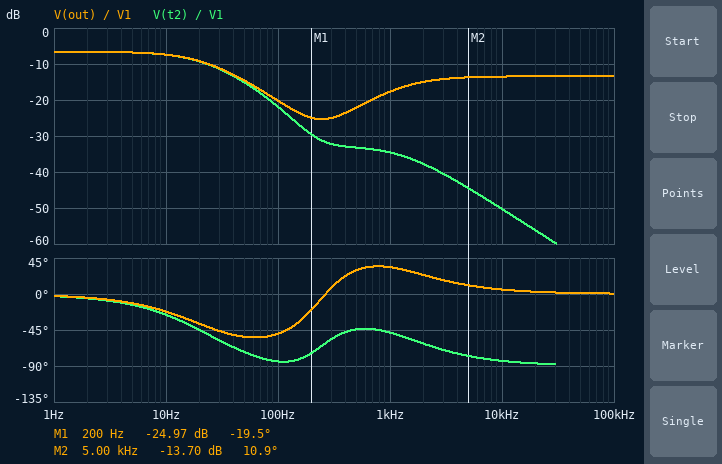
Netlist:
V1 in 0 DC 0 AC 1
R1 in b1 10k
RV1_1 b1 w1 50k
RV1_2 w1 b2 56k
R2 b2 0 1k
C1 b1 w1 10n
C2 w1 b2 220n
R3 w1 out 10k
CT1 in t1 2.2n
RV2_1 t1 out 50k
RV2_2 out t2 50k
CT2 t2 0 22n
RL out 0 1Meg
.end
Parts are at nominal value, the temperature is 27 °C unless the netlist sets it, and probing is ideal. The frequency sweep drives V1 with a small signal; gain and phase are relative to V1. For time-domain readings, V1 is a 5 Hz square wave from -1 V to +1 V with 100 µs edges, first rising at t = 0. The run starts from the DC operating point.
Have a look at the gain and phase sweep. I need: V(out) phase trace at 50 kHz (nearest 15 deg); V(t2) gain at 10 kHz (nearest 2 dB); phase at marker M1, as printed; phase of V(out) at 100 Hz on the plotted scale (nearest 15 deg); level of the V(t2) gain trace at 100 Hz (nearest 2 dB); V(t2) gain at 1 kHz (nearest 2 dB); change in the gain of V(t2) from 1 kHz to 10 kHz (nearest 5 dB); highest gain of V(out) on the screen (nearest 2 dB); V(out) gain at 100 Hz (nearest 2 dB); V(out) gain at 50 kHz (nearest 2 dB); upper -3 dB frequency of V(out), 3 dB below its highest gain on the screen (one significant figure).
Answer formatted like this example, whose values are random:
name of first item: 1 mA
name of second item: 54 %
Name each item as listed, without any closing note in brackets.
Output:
V(out) phase trace at 50 kHz: 0 deg
V(t2) gain at 10 kHz: -50 dB
phase at marker M1, as printed: -19.5 deg
phase of V(out) at 100 Hz on the plotted scale: -45 deg
level of the V(t2) gain trace at 100 Hz: -22 dB
V(t2) gain at 1 kHz: -34 dB
change in the gain of V(t2) from 1 kHz to 10 kHz: -15 dB
highest gain of V(out) on the screen: -6 dB
V(out) gain at 100 Hz: -20 dB
V(out) gain at 50 kHz: -14 dB
upper -3 dB frequency of V(out), 3 dB below its highest gain on the screen: 20 Hz
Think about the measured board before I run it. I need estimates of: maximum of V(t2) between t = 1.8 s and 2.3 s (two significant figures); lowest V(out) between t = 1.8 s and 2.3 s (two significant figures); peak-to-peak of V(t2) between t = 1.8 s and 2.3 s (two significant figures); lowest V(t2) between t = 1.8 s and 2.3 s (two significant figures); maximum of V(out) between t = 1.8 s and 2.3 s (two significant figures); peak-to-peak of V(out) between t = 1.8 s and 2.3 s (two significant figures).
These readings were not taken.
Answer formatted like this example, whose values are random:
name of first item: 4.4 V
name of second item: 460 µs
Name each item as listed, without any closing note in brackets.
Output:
maximum of V(t2) between t = 1.8 s and 2.3 s: 470 mV
lowest V(out) between t = 1.8 s and 2.3 s: -470 mV
peak-to-peak of V(t2) between t = 1.8 s and 2.3 s: 940 mV
lowest V(t2) between t = 1.8 s and 2.3 s: -470 mV
maximum of V(out) between t = 1.8 s and 2.3 s: 470 mV
peak-to-peak of V(out) between t = 1.8 s and 2.3 s: 940 mV
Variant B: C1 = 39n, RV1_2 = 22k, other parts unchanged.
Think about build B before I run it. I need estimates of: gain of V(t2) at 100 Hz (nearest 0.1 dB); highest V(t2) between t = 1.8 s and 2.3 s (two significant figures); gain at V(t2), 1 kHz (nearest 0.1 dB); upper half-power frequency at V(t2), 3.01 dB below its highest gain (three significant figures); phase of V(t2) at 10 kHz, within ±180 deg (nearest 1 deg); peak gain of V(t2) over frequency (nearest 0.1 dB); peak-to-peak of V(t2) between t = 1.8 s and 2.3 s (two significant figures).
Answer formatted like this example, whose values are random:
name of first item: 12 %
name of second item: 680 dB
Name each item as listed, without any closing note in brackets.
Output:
gain of V(t2) at 100 Hz: -18.8 dB
highest V(t2) between t = 1.8 s and 2.3 s: 270 mV
gain at V(t2), 1 kHz: -33.6 dB
upper half-power frequency at V(t2), 3.01 dB below its highest gain: 40.5 Hz
phase of V(t2) at 10 kHz, within ±180 deg: -85 deg
peak gain of V(t2) over frequency: -11.4 dB
peak-to-peak of V(t2) between t = 1.8 s and 2.3 s: 540 mV
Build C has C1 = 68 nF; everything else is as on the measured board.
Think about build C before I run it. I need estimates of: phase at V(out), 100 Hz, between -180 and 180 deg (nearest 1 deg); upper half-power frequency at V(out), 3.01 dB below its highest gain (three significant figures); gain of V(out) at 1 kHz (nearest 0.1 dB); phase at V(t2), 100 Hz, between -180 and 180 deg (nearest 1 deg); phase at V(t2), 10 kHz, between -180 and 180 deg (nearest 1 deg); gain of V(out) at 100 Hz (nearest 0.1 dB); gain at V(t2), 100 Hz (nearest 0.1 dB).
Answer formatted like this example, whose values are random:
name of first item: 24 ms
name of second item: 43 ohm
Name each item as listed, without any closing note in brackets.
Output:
phase at V(out), 100 Hz, between -180 and 180 deg: -23 deg
upper half-power frequency at V(out), 3.01 dB below its highest gain: 22.9 Hz
gain of V(out) at 1 kHz: -16.9 dB
phase at V(t2), 100 Hz, between -180 and 180 deg: -58 deg
phase at V(t2), 10 kHz, between -180 and 180 deg: -86 deg
gain of V(out) at 100 Hz: -14.3 dB
gain at V(t2), 100 Hz: -16.0 dB
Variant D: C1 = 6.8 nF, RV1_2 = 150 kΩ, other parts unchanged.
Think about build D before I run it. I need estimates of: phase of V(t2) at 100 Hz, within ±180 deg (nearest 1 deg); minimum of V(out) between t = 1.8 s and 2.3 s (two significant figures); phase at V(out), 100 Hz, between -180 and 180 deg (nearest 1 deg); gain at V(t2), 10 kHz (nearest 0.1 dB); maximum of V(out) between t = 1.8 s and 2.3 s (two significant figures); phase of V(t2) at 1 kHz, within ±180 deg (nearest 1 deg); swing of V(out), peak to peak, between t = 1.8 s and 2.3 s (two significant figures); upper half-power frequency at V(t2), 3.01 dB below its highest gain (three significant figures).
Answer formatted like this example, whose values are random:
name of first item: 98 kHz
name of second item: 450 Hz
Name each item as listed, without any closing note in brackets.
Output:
phase of V(t2) at 100 Hz, within ±180 deg: -93 deg
minimum of V(out) between t = 1.8 s and 2.3 s: -680 mV
phase at V(out), 100 Hz, between -180 and 180 deg: -58 deg
gain at V(t2), 10 kHz: -50.3 dB
maximum of V(out) between t = 1.8 s and 2.3 s: 680 mV
phase of V(t2) at 1 kHz, within ±180 deg: -46 deg
swing of V(out), peak to peak, between t = 1.8 s and 2.3 s: 1.4 V
upper half-power frequency at V(t2), 3.01 dB below its highest gain: 15.0 Hz
